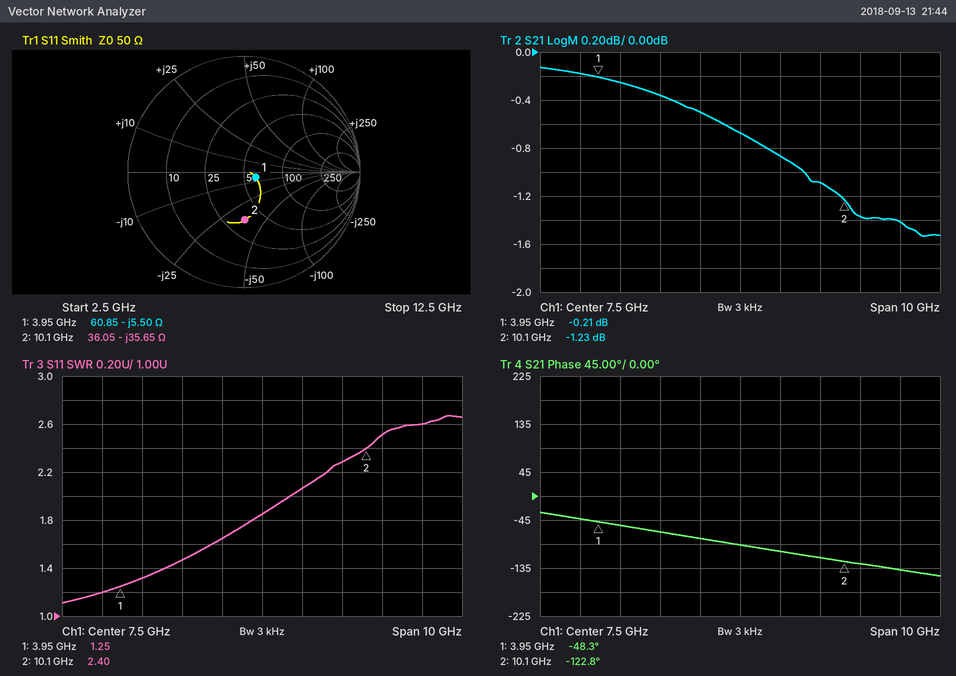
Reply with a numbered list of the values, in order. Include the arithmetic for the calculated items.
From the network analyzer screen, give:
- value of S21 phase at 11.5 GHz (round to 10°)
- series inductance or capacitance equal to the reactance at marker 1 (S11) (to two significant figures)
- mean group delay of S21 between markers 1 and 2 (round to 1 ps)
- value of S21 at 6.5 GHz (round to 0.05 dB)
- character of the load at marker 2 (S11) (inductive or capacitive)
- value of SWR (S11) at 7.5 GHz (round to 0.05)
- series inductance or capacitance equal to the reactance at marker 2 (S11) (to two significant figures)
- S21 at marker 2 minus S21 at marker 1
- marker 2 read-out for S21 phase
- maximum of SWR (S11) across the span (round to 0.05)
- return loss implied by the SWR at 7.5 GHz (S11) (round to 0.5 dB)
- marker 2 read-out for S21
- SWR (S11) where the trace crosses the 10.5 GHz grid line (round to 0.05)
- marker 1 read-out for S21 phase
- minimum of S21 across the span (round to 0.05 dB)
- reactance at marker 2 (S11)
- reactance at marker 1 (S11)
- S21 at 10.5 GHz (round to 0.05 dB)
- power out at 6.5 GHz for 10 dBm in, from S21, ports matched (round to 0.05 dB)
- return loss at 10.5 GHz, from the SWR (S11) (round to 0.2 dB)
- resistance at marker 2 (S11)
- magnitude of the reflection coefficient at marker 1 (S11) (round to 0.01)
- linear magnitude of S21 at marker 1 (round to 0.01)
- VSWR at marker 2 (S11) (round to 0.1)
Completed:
1. -140°
2. C = 1/(2π × 3.95 GHz × 5.5 Ω) ≈ 7.3 pF
3. −(-122.8° − (-48.3°))/(360° × 6.15 GHz) ≈ 34 ps
4. -0.50 dB
5. capacitive
6. 1.85
7. C = 1/(2π × 10.1 GHz × 35.65 Ω) ≈ 442 fF, so 440 fF to two significant figures
8. -1.23 − (-0.21) = -1.02 dB
9. -122.8°
10. 2.65
11. −20 log10((1.85 − 1)/(1.85 + 1)) ≈ 10.5 dB
12. -1.23 dB
13. 2.50
14. -48.3°
15. -1.55 dB
16. -35.65 Ω
17. -5.50 Ω
18. -1.35 dB
19. 10 dBm + (-0.50 dB) = 9.50 dBm
20. −20 log10((2.5 − 1)/(2.5 + 1)) ≈ 7.4 dB
21. 36.05 Ω
22. 0.11
23. 10^(-0.21/20) ≈ 0.98
24. 2.4
